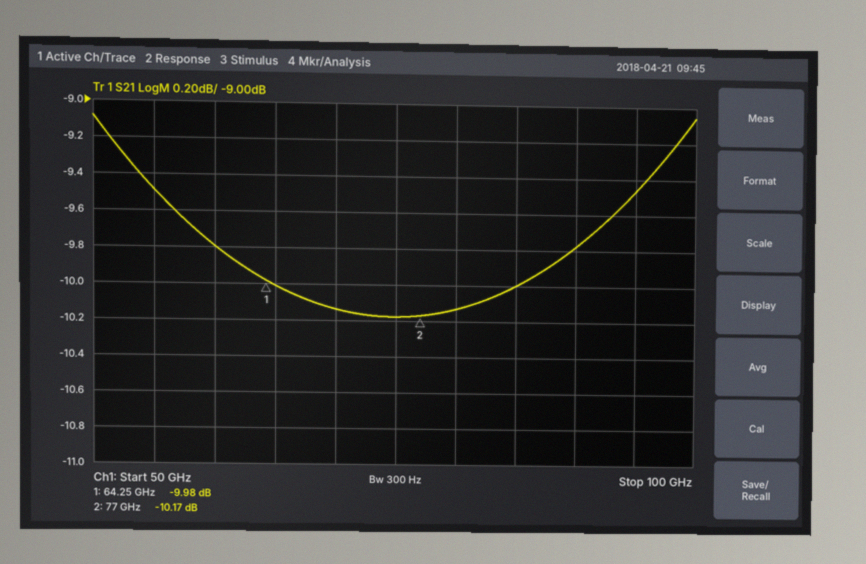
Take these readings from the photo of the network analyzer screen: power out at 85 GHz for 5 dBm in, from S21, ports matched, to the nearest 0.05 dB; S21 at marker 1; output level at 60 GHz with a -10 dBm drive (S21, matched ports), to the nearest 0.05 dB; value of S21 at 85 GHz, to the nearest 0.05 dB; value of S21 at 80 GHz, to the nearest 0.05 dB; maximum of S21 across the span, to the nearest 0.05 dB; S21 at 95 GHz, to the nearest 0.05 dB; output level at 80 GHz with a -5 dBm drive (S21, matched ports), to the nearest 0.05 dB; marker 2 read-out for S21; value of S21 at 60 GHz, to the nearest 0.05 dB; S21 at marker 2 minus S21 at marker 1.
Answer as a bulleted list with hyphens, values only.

- -5.00 dBm
- -9.98 dB
- -19.80 dBm
- -10.00 dB
- -10.15 dB
- -9.05 dB
- -9.45 dB
- -15.15 dBm
- -10.17 dB
- -9.80 dB
- -0.19 dB
